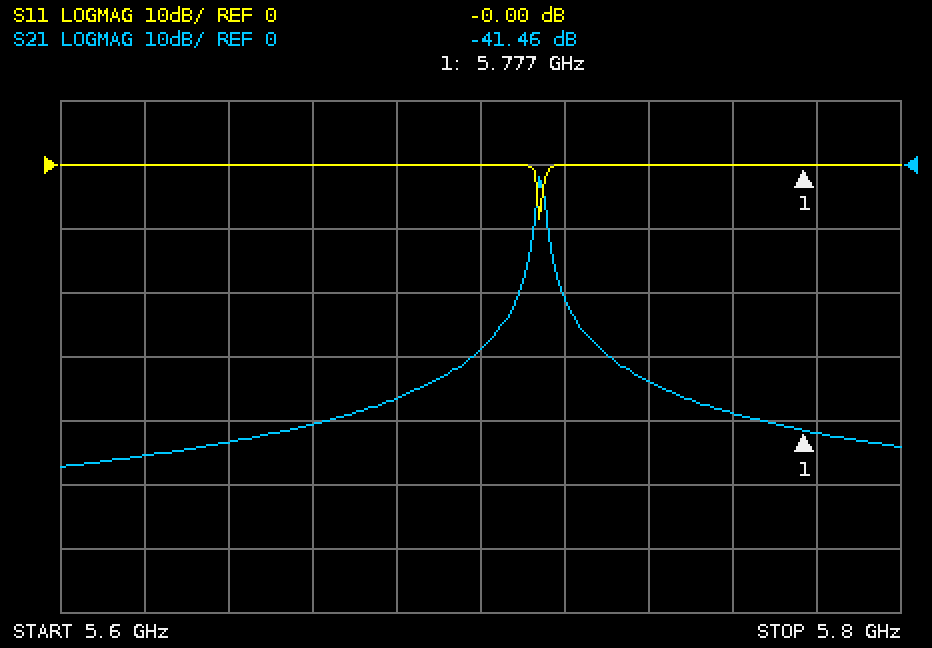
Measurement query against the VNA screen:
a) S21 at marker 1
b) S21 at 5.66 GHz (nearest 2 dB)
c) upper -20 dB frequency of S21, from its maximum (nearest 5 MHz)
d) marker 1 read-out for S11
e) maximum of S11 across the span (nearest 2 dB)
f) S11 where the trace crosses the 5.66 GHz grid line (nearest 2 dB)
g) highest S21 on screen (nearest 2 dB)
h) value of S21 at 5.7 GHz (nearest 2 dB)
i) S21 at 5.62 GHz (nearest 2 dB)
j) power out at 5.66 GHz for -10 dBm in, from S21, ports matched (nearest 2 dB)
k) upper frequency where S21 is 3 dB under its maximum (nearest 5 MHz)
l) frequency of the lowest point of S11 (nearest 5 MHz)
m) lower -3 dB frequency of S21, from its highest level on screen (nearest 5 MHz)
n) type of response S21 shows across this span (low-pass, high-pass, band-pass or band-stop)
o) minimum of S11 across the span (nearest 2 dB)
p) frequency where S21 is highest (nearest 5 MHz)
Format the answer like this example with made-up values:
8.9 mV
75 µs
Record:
-41.46 dB
-40 dB
5.720 GHz
-0.00 dB
0 dB
0 dB
-2 dB
-28 dB
-46 dB
-50 dBm
5.715 GHz
5.715 GHz
5.715 GHz
band-pass
-8 dB
5.715 GHz
